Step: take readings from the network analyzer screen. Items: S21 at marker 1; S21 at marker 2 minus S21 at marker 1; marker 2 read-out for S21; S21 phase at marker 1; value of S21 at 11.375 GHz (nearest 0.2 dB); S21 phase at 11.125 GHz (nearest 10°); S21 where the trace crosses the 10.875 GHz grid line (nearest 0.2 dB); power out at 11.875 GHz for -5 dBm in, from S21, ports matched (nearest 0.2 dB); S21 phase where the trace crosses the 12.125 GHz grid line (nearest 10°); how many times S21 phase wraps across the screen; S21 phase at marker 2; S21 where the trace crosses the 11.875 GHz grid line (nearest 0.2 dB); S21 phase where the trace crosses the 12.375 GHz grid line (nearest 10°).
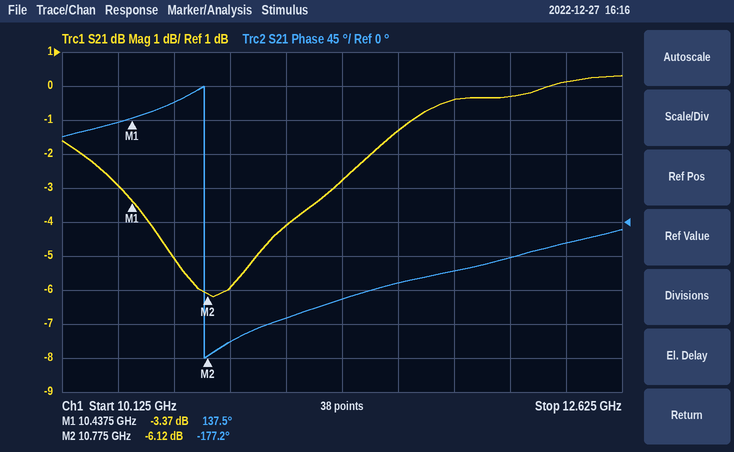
-3.37 dB
-2.75 dB
-6.12 dB
137.5°
-2.8 dB
-130°
-6.0 dB
-5.4 dBm
-50°
1
-177.2°
-0.4 dB
-30°
